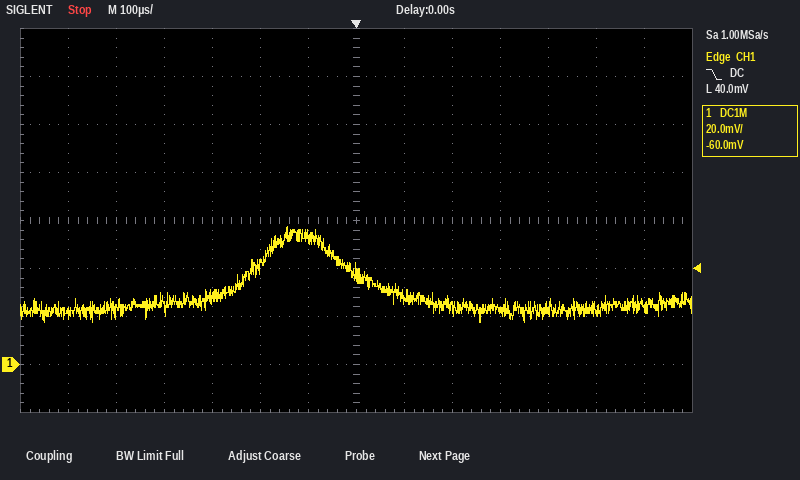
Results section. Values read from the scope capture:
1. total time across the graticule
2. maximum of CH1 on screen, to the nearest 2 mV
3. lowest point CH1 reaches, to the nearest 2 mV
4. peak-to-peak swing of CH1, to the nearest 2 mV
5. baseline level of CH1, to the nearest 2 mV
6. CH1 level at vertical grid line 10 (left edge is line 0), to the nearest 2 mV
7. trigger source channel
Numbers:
1.4 ms
58 mV
18 mV
40 mV
24 mV
22 mV
CH1
